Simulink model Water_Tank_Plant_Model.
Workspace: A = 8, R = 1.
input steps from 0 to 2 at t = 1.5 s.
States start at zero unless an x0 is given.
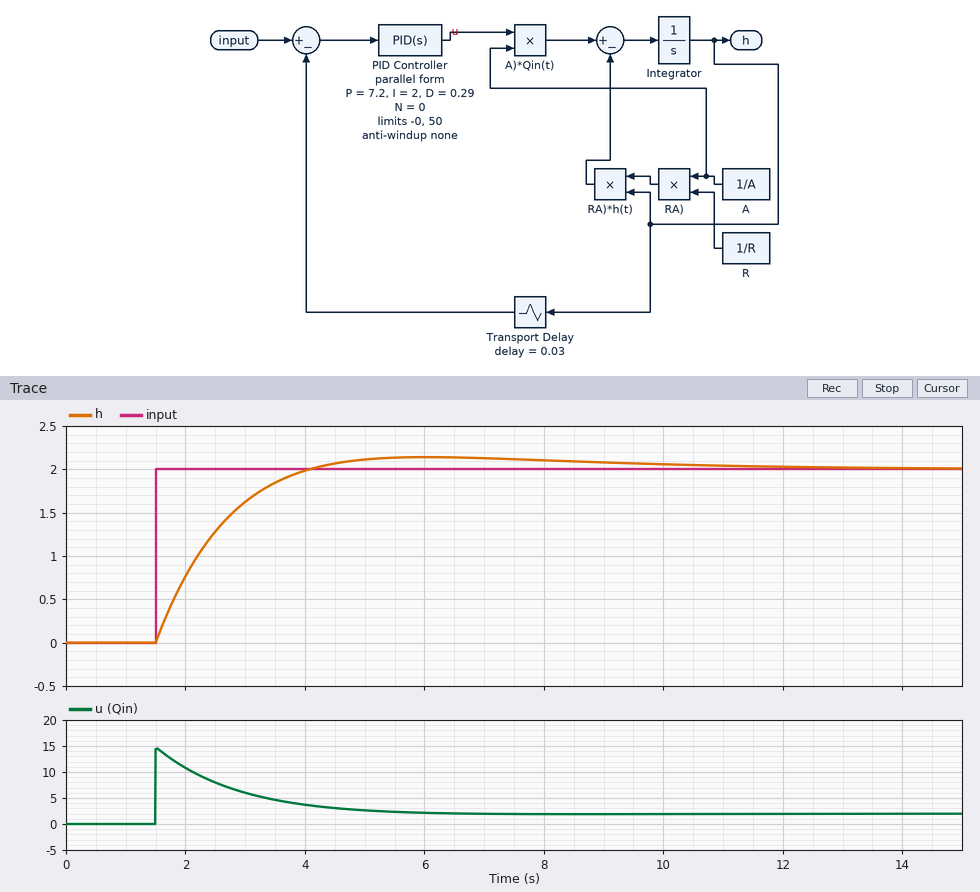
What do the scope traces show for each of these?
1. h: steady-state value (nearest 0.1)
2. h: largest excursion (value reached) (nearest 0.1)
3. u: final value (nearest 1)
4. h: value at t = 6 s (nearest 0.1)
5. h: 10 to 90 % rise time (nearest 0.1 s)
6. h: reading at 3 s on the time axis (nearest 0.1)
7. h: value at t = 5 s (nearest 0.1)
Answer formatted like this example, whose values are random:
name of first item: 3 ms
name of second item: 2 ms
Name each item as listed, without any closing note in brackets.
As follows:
h: steady-state value: 2.0
h: largest excursion (value reached): 2.1
u: final value: 2
h: value at t = 6 s: 2.1
h: 10 to 90 % rise time: 1.8 s
h: reading at 3 s on the time axis: 1.6
h: value at t = 5 s: 2.1
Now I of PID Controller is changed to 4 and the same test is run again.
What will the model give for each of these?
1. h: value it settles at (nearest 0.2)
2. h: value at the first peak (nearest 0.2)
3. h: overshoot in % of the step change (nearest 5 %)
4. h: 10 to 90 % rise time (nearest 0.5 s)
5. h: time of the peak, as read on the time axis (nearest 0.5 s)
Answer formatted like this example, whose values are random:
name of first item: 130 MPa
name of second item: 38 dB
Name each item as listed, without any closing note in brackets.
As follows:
h: value it settles at: 2.0
h: value at the first peak: 2.4
h: overshoot in % of the step change: 15 %
h: 10 to 90 % rise time: 1.5 s
h: time of the peak, as read on the time axis: 5.0 s
